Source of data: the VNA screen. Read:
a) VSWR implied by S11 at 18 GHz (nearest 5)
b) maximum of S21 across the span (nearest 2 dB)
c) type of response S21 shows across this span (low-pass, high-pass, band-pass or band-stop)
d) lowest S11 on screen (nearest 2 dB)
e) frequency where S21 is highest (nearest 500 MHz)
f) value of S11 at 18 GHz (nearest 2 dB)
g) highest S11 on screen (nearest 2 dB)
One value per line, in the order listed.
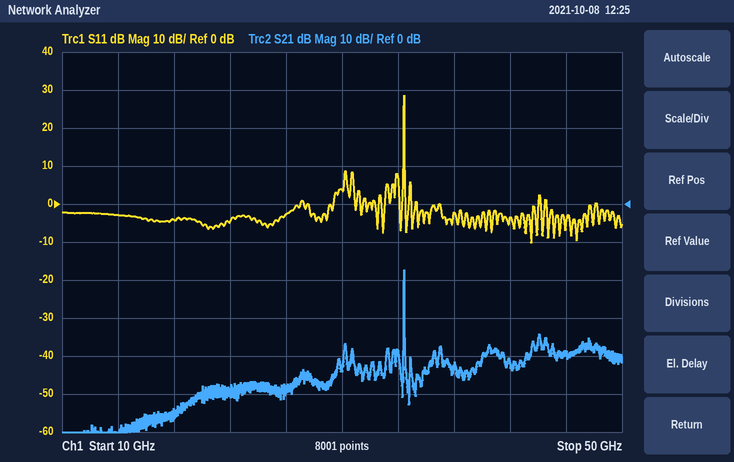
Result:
5
-18 dB
band-pass
-10 dB
34.5 GHz
-4 dB
28 dB
